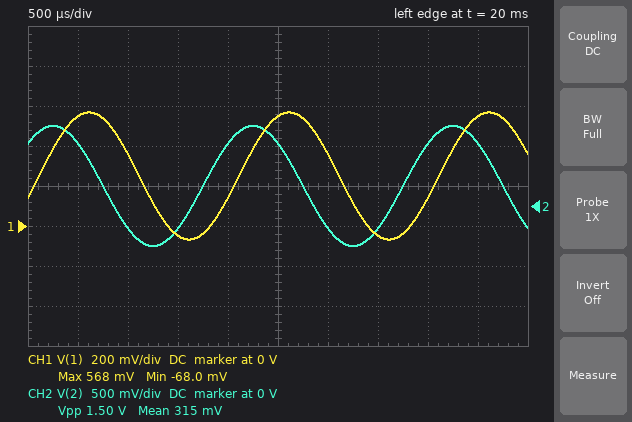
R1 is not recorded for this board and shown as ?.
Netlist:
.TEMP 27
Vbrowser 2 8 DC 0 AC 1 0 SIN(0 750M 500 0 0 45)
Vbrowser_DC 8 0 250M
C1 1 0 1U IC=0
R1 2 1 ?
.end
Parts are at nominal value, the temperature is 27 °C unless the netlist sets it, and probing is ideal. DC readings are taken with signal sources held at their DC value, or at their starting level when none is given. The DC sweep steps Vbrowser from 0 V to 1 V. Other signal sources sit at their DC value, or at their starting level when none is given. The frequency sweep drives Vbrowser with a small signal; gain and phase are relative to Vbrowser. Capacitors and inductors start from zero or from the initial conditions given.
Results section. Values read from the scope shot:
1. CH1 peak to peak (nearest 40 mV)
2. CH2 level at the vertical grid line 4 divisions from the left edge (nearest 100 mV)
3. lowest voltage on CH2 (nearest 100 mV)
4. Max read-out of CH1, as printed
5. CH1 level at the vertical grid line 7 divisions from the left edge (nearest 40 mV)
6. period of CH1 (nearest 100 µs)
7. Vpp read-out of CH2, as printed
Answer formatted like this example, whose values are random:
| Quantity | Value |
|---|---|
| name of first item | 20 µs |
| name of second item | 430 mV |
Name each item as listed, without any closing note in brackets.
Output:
| Quantity | Value |
|---|---|
| CH1 peak to peak | 640 mV |
| CH2 level at the vertical grid line 4 divisions from the left edge | 800 mV |
| lowest voltage on CH2 | -500 mV |
| Max read-out of CH1, as printed | 568 mV |
| CH1 level at the vertical grid line 7 divisions from the left edge | -40 mV |
| period of CH1 | 2.0 ms |
| Vpp read-out of CH2, as printed | 1.50 V |
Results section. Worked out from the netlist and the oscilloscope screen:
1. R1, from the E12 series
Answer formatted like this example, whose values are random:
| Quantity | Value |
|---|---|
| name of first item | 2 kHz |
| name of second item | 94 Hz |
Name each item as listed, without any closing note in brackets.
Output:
| Quantity | Value |
|---|---|
| R1, from the E12 series | 680 Ω |
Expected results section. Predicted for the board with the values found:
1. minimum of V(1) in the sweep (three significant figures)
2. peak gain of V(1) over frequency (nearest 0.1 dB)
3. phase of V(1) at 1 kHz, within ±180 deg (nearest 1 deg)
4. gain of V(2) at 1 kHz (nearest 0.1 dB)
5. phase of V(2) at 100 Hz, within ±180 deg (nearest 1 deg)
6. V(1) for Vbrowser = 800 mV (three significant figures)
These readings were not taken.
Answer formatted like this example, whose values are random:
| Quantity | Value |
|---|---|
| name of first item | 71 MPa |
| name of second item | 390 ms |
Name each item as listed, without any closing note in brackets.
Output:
| Quantity | Value |
|---|---|
| minimum of V(1) in the sweep | 250 mV |
| peak gain of V(1) over frequency | 0 dB |
| phase of V(1) at 1 kHz, within ±180 deg | -77 deg |
| gain of V(2) at 1 kHz | 0 dB |
| phase of V(2) at 100 Hz, within ±180 deg | 0 deg |
| V(1) for Vbrowser = 800 mV | 1.05 V |
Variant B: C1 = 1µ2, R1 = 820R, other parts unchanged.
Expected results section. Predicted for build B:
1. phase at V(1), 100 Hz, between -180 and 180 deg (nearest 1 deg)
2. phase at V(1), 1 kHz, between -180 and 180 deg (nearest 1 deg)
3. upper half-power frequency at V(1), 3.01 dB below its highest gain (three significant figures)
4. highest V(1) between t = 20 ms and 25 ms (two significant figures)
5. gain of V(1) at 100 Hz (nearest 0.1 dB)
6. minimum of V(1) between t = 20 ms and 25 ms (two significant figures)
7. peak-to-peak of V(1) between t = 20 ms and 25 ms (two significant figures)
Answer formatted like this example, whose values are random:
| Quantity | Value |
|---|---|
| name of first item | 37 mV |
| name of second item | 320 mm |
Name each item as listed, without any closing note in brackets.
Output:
| Quantity | Value |
|---|---|
| phase at V(1), 100 Hz, between -180 and 180 deg | -32 deg |
| phase at V(1), 1 kHz, between -180 and 180 deg | -81 deg |
| upper half-power frequency at V(1), 3.01 dB below its highest gain | 162 Hz |
| highest V(1) between t = 20 ms and 25 ms | 480 mV |
| gain of V(1) at 100 Hz | -1.4 dB |
| minimum of V(1) between t = 20 ms and 25 ms | 19 mV |
| peak-to-peak of V(1) between t = 20 ms and 25 ms | 460 mV |
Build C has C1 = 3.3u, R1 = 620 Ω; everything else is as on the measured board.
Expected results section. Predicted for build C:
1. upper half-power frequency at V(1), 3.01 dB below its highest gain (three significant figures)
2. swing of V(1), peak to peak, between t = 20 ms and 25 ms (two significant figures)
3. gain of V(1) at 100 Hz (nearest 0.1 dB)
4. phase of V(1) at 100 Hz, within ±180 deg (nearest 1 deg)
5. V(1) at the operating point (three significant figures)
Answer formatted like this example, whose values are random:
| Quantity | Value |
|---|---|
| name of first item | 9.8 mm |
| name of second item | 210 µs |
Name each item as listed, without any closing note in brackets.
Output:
| Quantity | Value |
|---|---|
| upper half-power frequency at V(1), 3.01 dB below its highest gain | 77.8 Hz |
| swing of V(1), peak to peak, between t = 20 ms and 25 ms | 230 mV |
| gain of V(1) at 100 Hz | -4.2 dB |
| phase of V(1) at 100 Hz, within ±180 deg | -52 deg |
| V(1) at the operating point | 250 mV |
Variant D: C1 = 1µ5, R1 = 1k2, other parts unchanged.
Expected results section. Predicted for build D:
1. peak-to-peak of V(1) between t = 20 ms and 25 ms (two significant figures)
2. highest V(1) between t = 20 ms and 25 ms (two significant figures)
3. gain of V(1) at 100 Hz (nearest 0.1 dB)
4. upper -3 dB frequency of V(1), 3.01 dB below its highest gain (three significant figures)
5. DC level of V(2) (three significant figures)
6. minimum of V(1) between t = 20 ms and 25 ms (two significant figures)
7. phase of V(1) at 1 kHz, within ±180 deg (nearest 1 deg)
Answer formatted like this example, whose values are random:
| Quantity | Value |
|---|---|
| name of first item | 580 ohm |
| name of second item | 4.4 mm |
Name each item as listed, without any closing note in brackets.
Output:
| Quantity | Value |
|---|---|
| peak-to-peak of V(1) between t = 20 ms and 25 ms | 260 mV |
| highest V(1) between t = 20 ms and 25 ms | 380 mV |
| gain of V(1) at 100 Hz | -3.6 dB |
| upper -3 dB frequency of V(1), 3.01 dB below its highest gain | 88.4 Hz |
| DC level of V(2) | 250 mV |
| minimum of V(1) between t = 20 ms and 25 ms | 120 mV |
| phase of V(1) at 1 kHz, within ±180 deg | -85 deg |
